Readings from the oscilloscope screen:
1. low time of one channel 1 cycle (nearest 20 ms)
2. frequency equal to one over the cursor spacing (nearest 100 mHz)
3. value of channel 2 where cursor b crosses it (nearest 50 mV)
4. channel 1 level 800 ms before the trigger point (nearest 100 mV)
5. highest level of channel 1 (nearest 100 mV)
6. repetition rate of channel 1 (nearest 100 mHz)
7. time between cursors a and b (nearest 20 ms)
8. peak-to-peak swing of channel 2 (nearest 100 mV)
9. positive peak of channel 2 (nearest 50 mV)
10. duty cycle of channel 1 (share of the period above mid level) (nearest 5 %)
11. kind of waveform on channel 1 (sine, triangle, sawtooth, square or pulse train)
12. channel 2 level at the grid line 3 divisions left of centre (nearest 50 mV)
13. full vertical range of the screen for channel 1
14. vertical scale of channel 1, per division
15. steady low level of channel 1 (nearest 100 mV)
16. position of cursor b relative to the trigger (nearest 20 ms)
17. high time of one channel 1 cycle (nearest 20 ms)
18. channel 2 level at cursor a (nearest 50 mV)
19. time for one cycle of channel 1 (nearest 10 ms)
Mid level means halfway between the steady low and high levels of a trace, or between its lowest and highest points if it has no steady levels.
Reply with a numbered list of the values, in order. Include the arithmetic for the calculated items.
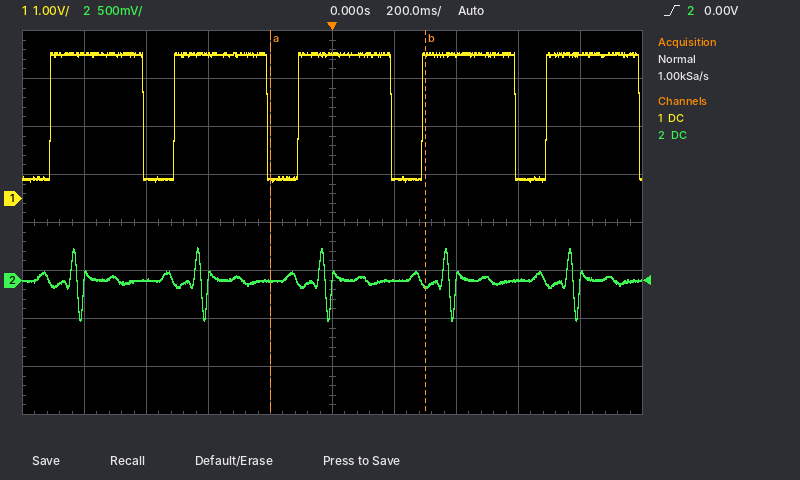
1. 100 ms
2. 1 / 500 ms ≈ 2.0 Hz
3. -50 mV
4. 3.0 V
5. 3.0 V
6. 1 / 400 ms ≈ 2.5 Hz
7. 500 ms
8. 800 mV
9. 350 mV
10. 300 ms / 400 ms ≈ 75 %
11. pulse train
12. 0 mV
13. 8 V
14. 1 V
15. 400 mV
16. +300 ms
17. 300 ms
18. 0 mV
19. 400 ms
